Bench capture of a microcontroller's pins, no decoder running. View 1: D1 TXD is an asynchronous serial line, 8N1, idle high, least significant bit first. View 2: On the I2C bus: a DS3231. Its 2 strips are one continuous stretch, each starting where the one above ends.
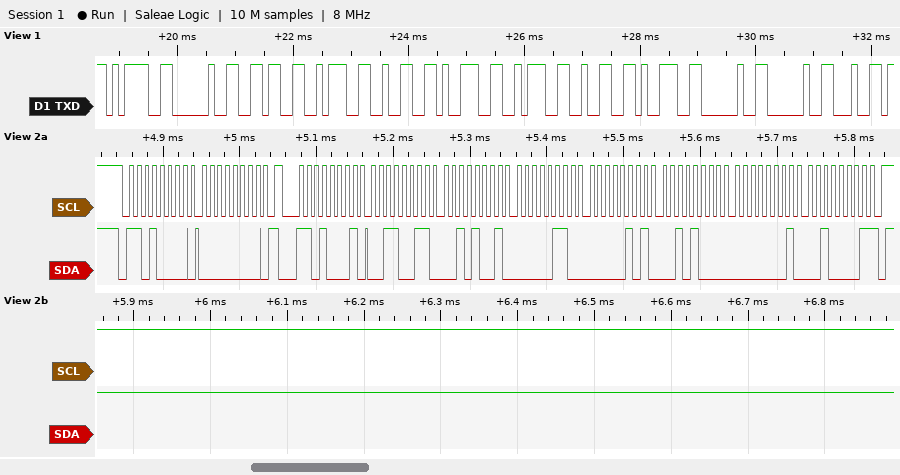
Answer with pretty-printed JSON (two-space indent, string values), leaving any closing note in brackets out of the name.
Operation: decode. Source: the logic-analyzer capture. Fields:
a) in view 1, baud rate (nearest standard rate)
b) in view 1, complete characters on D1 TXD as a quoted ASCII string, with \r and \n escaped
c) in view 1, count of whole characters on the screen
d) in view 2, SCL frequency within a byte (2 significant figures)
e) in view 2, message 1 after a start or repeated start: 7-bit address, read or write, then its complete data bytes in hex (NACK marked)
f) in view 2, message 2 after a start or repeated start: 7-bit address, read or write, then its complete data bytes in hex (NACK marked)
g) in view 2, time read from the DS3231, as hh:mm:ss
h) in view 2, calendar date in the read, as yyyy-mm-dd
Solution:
{
  "in view 1, baud rate": "9600 baud",
  "in view 1, complete characters on D1 TXD as a quoted ASCII string, with \\r and \\n escaped": "\"= 6:29:29  d\"",
  "in view 1, count of whole characters on the screen": "12",
  "in view 2, SCL frequency within a byte": "100 kHz",
  "in view 2, message 1 after a start or repeated start: 7-bit address, read or write, then its complete data bytes in hex": "0x68 write: 00",
  "in view 2, message 2 after a start or repeated start: 7-bit address, read or write, then its complete data bytes in hex": "0x68 read: 33 29 06 05 28 01 21 NACK",
  "in view 2, time read from the DS3231, as hh:mm:ss": "06:29:33",
  "in view 2, calendar date in the read, as yyyy-mm-dd": "2021-01-28"
}
